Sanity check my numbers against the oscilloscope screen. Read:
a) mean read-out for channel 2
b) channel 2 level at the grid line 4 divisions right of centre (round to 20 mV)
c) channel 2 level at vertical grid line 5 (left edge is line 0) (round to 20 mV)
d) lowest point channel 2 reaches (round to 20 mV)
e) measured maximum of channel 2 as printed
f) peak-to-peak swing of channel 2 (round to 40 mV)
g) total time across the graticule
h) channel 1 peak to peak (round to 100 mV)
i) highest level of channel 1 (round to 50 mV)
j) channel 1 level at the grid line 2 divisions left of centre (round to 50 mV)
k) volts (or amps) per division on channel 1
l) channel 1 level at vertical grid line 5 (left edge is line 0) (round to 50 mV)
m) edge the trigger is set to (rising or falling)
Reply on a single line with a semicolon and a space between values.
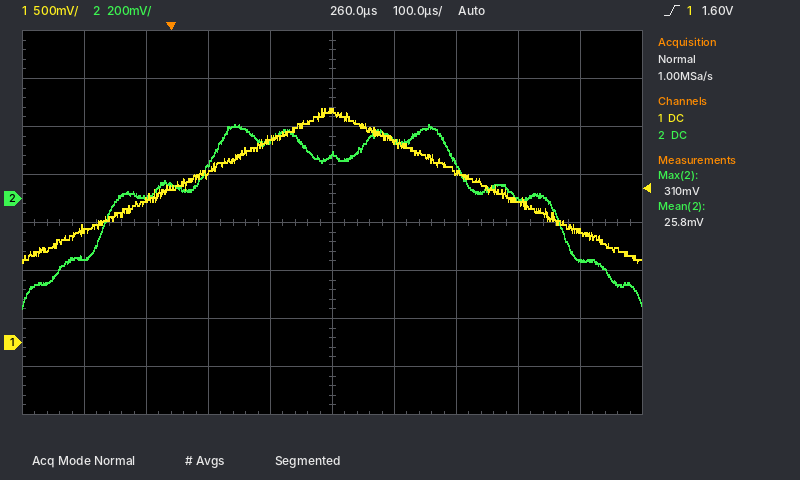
25.8 mV; -260 mV; 180 mV; -460 mV; 310 mV; 760 mV; 1 ms; 1.60 V; 2.45 V; 1.75 V; 500 mV; 2.40 V; rising
